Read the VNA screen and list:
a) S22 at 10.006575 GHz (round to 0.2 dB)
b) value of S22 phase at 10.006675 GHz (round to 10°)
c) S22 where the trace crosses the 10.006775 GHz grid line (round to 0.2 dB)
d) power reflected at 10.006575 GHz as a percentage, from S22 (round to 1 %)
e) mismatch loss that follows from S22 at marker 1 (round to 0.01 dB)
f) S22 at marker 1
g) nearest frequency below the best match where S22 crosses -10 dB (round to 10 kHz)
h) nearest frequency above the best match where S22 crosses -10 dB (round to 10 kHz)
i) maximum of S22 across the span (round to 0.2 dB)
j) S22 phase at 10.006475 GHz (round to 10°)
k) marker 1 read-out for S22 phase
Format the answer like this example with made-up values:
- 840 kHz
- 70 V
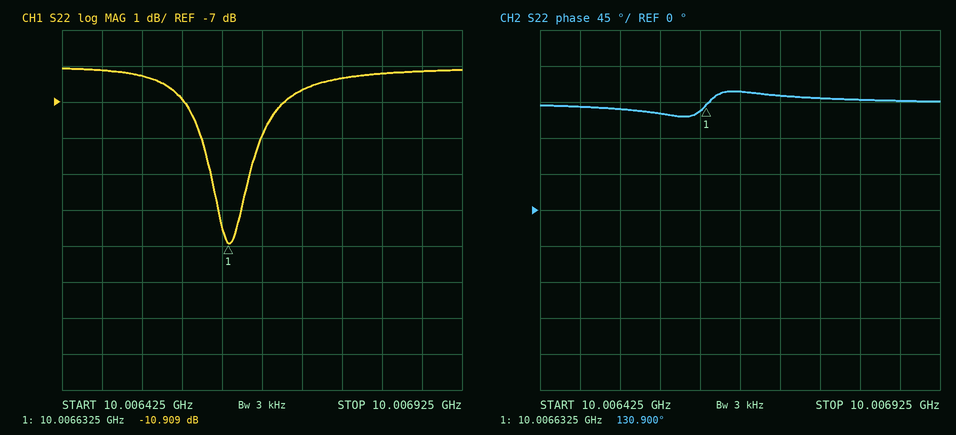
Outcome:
- -7.0 dB
- 150°
- -6.4 dB
- 20 %
- 0.37 dB
- -10.909 dB
- 10.00662 GHz
- 10.00665 GHz
- -6.0 dB
- 130°
- 130.900°
